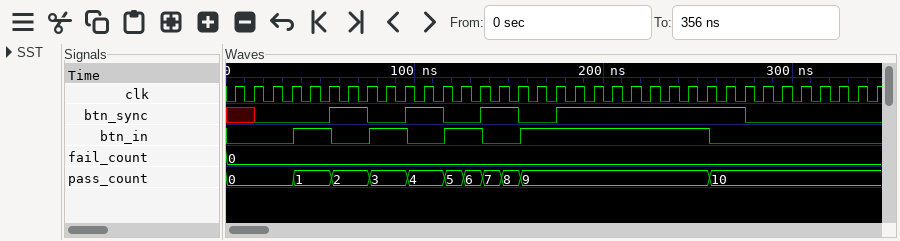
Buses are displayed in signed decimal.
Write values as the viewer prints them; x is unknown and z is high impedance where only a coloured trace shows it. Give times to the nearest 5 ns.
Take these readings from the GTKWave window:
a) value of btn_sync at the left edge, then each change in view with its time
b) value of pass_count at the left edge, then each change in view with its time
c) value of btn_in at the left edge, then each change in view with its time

x, 0 at 15 ns, 1 at 55 ns, 0 at 75 ns, 1 at 95 ns, 0 at 115 ns, 1 at 135 ns, 0 at 155 ns, 1 at 175 ns, 0 at 275 ns
0, 1 at 35 ns, 2 at 55 ns, 3 at 75 ns, 4 at 95 ns, 5 at 115 ns, 6 at 125 ns, 7 at 135 ns, 8 at 145 ns, 9 at 155 ns, 10 at 255 ns
0, 1 at 35 ns, 0 at 55 ns, 1 at 75 ns, 0 at 95 ns, 1 at 115 ns, 0 at 135 ns, 1 at 155 ns, 0 at 255 ns
